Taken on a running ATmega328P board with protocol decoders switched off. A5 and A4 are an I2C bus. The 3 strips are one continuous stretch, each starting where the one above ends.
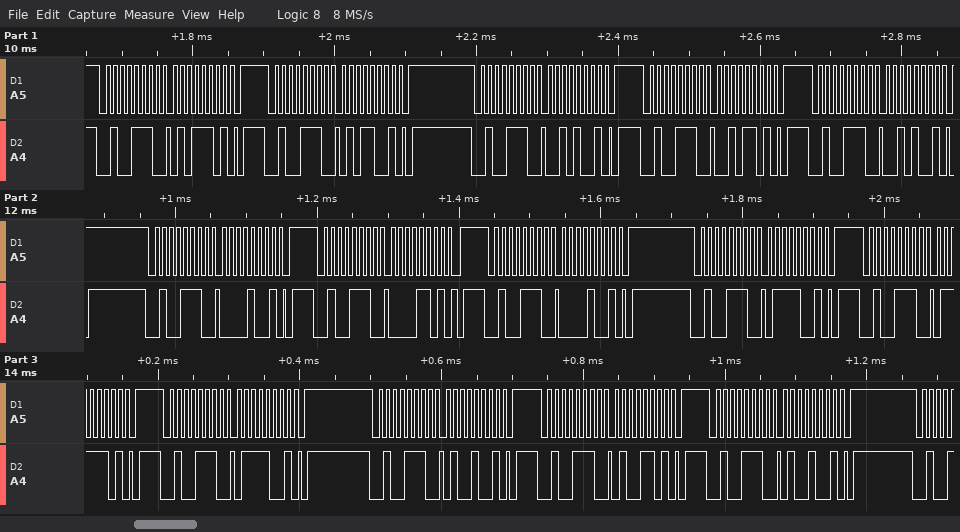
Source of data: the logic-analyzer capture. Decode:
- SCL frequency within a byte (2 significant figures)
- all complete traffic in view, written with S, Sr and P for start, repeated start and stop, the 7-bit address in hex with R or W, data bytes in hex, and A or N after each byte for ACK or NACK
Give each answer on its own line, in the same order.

100 kHz
S 27W A 5D A P S 27W A 59 A P S 27W A 29 A P S 27W A 2D A P S 27W A 29 A P S 27W A 09 A P S 27W A 0D A P S 27W A 09 A P S 27W A 79 A P S 27W A 7D A P S 27W A 79 A P S 27W A 49 A P S 27W A 4D A P S 27W A 49 A P
